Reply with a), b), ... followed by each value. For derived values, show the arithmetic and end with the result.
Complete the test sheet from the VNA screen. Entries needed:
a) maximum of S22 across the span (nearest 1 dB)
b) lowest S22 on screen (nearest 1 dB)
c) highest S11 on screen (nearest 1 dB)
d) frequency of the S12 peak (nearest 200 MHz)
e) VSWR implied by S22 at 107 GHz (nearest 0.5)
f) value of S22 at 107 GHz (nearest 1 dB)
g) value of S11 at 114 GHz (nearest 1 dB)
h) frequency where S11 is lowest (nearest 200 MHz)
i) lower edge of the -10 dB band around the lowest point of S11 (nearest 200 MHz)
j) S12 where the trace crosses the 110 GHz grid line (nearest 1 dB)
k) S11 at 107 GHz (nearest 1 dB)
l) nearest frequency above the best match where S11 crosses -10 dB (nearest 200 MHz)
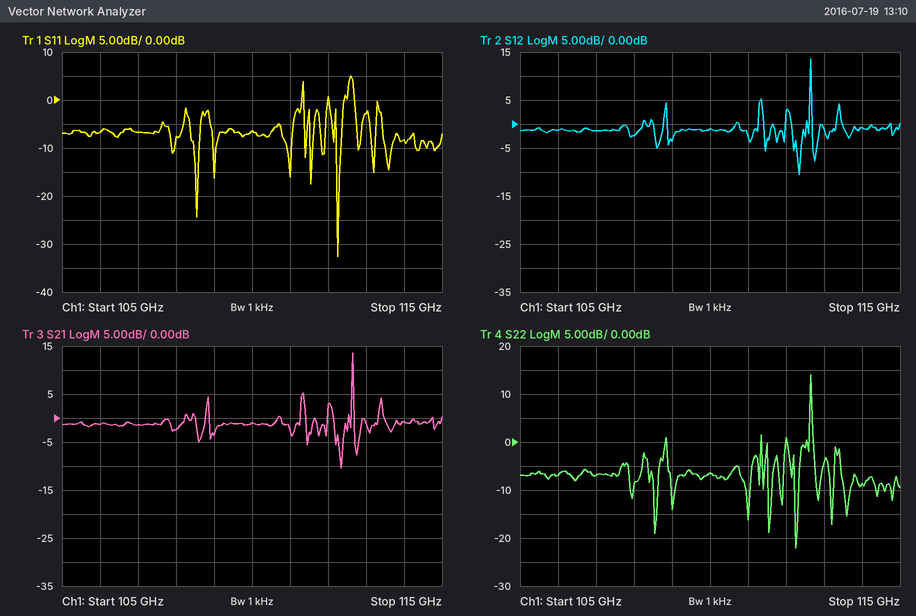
a) 14 dB
b) -22 dB
c) 5 dB
d) 112.6 GHz
e) |Γ| = 10^(-7/20) = 0.4467; VSWR = (1 + 0.4467)/(1 − 0.4467) ≈ 2.61, so 2.5 to the nearest 0.5
f) -7 dB
g) -8 dB
h) 112.2 GHz
i) 112.2 GHz
j) -1 dB
k) -7 dB
l) 112.4 GHz
